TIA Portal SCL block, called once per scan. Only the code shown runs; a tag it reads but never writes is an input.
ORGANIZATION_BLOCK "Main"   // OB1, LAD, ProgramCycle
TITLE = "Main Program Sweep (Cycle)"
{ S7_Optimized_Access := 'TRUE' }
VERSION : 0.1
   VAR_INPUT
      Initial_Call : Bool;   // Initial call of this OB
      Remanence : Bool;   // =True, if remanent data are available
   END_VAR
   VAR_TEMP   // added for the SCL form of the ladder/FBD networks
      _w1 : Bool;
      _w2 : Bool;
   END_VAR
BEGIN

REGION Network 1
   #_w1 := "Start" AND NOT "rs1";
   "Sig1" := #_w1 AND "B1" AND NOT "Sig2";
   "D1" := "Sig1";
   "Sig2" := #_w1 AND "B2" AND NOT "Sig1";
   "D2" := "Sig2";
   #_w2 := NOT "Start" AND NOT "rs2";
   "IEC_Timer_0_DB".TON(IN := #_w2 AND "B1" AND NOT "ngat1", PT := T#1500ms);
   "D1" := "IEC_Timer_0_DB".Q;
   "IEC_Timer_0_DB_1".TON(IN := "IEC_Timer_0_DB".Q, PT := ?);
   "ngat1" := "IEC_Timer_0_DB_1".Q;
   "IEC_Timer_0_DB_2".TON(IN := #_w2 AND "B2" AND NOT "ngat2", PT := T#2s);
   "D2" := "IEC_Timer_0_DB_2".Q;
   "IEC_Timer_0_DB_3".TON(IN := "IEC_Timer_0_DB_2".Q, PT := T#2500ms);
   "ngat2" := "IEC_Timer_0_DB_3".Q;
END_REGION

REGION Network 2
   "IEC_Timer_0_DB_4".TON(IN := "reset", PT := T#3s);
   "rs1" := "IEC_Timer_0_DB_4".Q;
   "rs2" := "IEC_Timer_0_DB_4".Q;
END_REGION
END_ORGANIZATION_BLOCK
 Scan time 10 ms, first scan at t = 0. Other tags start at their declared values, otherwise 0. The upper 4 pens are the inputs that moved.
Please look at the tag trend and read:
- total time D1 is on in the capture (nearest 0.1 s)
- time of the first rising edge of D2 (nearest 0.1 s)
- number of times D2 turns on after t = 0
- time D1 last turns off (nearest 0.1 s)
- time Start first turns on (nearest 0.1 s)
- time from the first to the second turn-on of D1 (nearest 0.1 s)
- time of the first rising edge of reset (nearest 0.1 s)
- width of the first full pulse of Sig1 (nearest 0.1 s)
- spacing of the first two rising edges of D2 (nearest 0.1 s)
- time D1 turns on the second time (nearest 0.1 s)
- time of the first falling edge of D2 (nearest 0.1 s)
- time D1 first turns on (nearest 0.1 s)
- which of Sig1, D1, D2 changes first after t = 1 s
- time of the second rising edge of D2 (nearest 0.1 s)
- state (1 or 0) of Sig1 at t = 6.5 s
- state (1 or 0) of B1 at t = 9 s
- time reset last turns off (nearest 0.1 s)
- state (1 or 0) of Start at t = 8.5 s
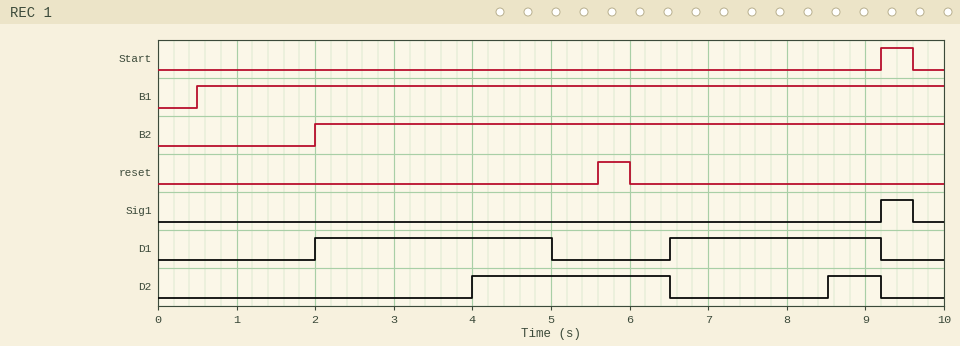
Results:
5.7 s
4.0 s
2
9.2 s
9.2 s
4.5 s
5.6 s
0.4 s
4.5 s
6.5 s
6.5 s
2.0 s
D1
8.5 s
0
1
6.0 s
0
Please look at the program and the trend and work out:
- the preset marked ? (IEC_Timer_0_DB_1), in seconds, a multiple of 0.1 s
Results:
3.0 s
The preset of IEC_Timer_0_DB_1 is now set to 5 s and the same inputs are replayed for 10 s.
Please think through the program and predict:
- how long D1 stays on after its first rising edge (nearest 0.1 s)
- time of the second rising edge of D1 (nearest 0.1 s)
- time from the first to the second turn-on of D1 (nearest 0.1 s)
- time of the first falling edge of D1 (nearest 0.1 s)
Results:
5.0 s
8.5 s
6.5 s
7.0 s
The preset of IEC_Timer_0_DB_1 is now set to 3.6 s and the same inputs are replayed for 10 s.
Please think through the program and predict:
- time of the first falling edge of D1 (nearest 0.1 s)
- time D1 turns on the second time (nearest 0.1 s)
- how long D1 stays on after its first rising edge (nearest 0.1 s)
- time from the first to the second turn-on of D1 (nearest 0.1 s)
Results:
5.6 s
7.1 s
3.6 s
5.1 s
